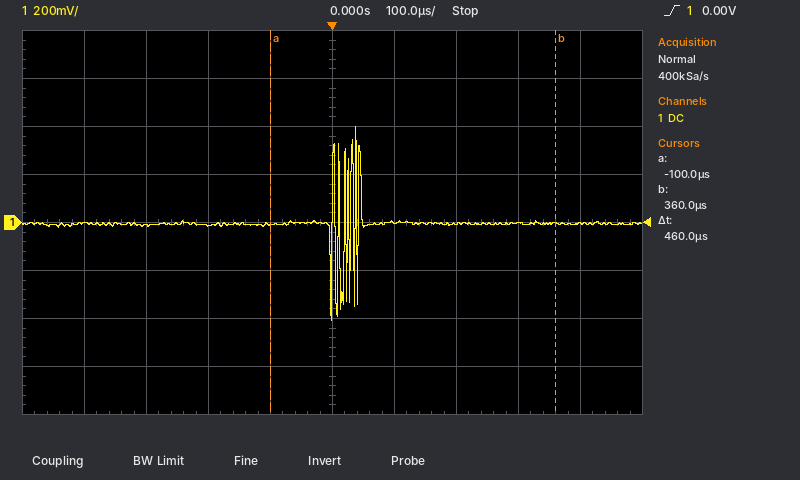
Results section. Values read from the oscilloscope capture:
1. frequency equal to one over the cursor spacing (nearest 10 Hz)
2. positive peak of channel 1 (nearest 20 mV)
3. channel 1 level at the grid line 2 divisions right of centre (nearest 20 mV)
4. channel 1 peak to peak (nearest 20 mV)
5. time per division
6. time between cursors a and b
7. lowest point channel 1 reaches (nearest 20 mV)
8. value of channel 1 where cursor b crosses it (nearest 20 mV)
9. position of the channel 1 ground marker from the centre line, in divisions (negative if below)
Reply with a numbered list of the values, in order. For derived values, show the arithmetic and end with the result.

1. 1 / 460 µs ≈ 2.17 kHz
2. 400 mV
3. 0 mV
4. 400 mV − (-400 mV) = 800 mV
5. 100 µs
6. 460 µs
7. -400 mV
8. 0 mV
9. 0.0 div
